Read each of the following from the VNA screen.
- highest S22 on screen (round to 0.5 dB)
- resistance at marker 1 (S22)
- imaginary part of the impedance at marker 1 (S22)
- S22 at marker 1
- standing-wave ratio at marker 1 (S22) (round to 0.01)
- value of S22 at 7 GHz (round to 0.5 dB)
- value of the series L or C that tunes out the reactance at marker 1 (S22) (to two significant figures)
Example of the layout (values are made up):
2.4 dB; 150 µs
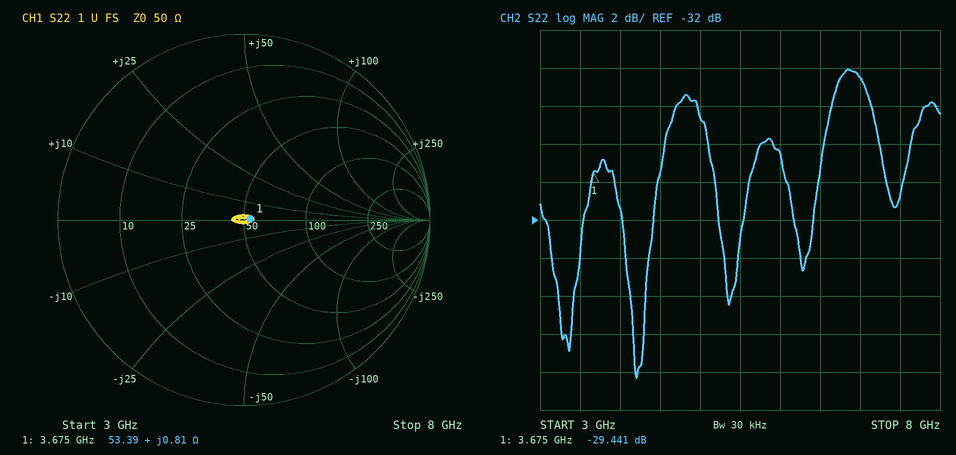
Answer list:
-24.0 dB; 53.39 Ω; +0.81 Ω; -29.441 dB; 1.07; -24.5 dB; 53 pF
